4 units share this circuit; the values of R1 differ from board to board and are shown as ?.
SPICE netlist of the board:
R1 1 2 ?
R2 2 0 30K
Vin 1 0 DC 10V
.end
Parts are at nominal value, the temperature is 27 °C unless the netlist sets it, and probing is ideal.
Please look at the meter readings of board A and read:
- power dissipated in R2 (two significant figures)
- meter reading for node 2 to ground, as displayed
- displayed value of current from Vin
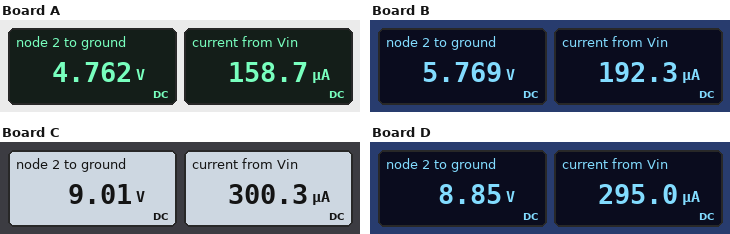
760 µW
4.762 V
158.7 µA
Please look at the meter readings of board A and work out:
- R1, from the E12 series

33 kΩ
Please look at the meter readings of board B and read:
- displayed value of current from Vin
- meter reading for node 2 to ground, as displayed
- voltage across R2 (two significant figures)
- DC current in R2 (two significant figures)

192.3 µA
5.769 V
5.8 V
190 µA
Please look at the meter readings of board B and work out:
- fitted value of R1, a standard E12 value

22 kΩ
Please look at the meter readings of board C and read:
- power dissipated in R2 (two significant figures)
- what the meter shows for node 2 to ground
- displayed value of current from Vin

2.7 mW
9.01 V
300.3 µA
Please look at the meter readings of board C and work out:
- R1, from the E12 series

3.3 kΩ
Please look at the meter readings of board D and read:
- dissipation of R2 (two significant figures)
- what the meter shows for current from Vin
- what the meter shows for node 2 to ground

2.6 mW
295.0 µA
8.85 V
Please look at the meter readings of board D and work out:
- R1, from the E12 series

3.9 kΩ
